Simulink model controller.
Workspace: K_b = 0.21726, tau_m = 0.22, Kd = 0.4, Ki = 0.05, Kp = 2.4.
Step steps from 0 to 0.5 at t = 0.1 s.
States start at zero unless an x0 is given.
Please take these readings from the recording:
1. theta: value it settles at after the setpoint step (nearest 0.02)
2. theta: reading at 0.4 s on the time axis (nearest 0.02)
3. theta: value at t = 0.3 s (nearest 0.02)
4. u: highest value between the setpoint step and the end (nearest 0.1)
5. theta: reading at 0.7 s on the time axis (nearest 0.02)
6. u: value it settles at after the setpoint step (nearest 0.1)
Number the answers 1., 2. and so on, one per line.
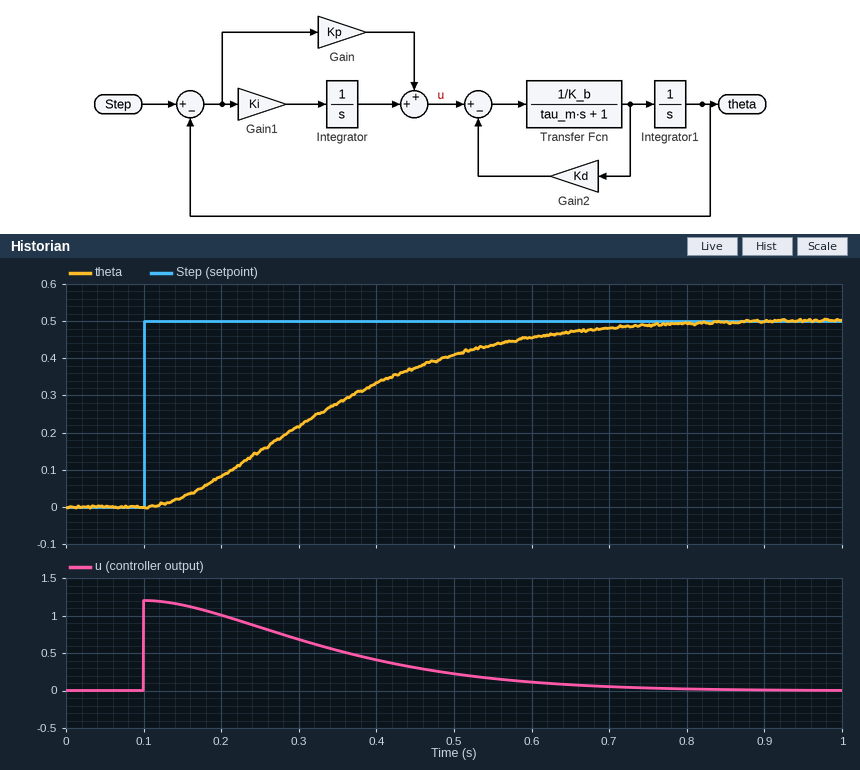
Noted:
1. 0.50
2. 0.34
3. 0.22
4. 1.2
5. 0.48
6. 0.0
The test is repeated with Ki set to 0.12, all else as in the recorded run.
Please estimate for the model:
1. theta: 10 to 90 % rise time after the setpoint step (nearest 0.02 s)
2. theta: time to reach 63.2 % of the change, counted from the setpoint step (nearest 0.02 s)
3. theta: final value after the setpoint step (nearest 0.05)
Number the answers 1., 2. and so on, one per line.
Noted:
1. 0.42 s
2. 0.28 s
3. 0.50
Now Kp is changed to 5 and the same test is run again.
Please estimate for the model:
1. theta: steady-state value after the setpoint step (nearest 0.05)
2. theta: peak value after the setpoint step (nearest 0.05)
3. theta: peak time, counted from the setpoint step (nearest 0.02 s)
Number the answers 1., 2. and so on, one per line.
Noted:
1. 0.50
2. 0.55
3. 0.40 s
